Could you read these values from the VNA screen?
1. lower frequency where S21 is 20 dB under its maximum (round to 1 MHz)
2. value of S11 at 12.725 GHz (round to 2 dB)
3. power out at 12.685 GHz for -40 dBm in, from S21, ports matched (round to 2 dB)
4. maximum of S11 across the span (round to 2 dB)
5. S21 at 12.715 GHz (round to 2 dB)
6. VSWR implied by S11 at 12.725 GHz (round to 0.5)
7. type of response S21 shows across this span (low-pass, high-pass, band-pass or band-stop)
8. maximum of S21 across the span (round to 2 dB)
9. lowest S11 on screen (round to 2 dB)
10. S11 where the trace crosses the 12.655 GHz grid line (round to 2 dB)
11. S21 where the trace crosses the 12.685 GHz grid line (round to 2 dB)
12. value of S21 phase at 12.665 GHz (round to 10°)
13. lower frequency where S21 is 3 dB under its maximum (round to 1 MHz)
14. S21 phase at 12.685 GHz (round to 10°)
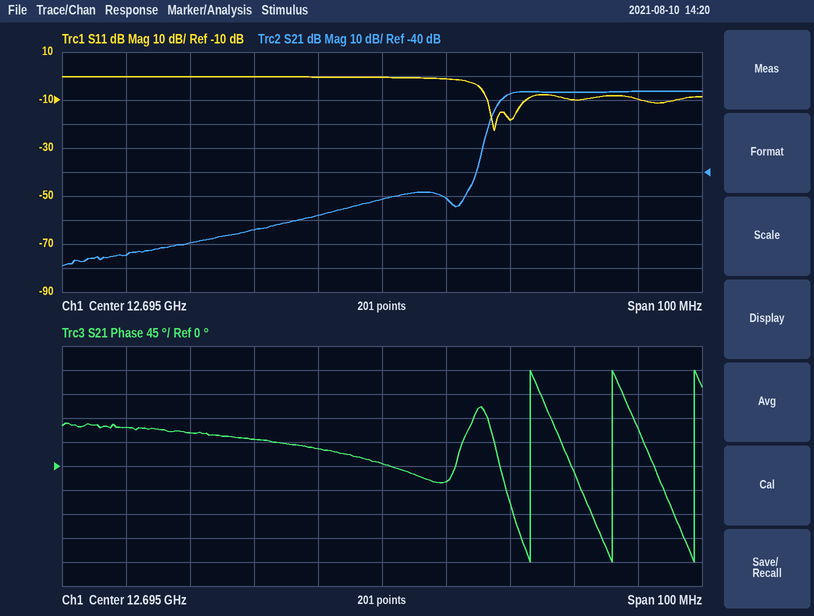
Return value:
12.711 GHz
-10 dB
-98 dBm
0 dB
-8 dB
2.0
high-pass
-6 dB
-22 dB
0 dB
-58 dB
60°
12.714 GHz
30°
